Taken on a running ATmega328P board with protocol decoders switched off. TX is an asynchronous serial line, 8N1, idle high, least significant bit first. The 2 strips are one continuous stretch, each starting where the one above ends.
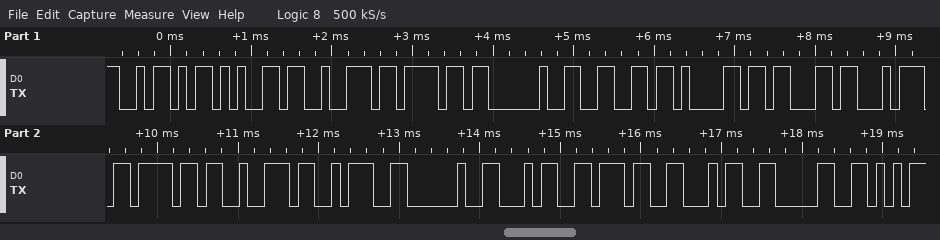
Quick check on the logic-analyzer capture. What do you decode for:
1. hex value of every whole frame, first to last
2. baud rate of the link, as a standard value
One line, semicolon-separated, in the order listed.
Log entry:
5A 65 72 6F 20 66 61 63 74 6F 72 3A 20 34 37 34 30; 9600 baud
